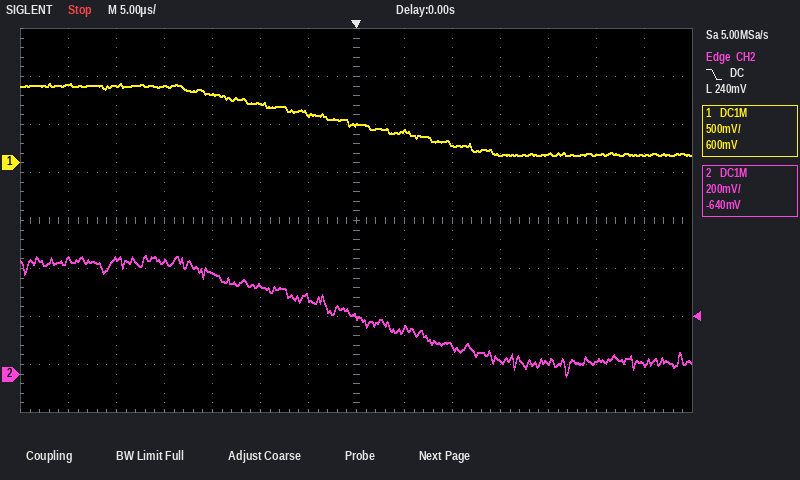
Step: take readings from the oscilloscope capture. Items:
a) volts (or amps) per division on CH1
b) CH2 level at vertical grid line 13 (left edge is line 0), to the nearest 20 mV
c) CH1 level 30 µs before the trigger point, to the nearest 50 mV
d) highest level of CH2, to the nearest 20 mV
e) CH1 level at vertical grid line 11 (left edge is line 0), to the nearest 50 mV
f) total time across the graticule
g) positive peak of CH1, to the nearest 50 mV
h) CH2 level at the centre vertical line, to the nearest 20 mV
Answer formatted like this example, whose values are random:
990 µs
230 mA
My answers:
500 mV
40 mV
800 mV
500 mV
100 mV
70 µs
850 mV
240 mV
